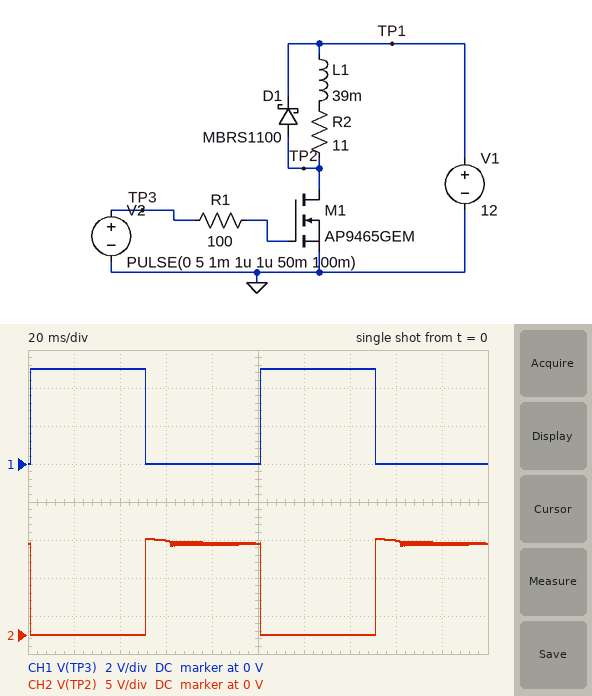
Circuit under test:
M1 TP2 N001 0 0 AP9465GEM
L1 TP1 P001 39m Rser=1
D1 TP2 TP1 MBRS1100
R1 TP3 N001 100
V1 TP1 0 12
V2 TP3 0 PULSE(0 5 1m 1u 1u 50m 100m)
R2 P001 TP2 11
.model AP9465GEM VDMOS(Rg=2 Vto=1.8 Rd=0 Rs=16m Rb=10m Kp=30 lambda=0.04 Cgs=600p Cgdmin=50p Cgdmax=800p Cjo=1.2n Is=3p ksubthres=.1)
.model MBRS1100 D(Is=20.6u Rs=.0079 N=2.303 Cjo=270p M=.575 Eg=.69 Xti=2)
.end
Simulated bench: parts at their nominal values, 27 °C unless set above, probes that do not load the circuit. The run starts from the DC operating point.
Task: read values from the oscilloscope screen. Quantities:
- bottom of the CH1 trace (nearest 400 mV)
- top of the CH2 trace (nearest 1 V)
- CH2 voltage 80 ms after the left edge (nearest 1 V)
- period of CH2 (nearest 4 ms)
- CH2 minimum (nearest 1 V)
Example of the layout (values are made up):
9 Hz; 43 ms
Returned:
0 V; 13 V; 12 V; 100 ms; 0 V
